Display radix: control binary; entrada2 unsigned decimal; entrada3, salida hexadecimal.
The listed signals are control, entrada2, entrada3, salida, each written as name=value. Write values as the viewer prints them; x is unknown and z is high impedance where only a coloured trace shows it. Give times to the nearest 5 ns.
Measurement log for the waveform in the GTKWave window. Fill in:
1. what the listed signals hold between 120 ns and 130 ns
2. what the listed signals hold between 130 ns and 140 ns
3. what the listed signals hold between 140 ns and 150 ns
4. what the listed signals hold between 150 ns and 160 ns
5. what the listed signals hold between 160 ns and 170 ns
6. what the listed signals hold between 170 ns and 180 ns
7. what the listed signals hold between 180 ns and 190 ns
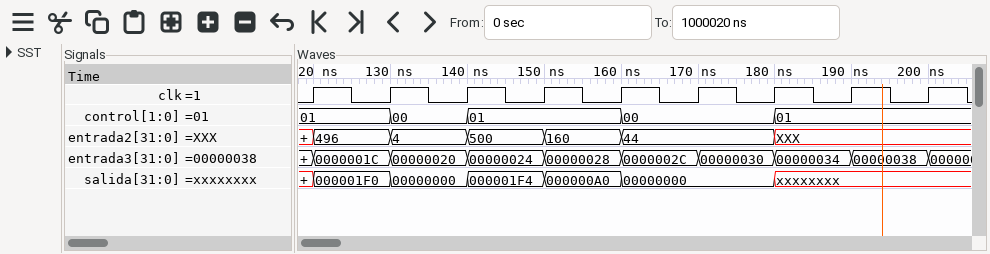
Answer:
control=01, entrada2=496, entrada3=0000001C, salida=000001F0
control=00, entrada2=4, entrada3=00000020, salida=00000000
control=01, entrada2=500, entrada3=00000024, salida=000001F4
control=01, entrada2=160, entrada3=00000028, salida=000000A0
control=00, entrada2=44, entrada3=0000002C, salida=00000000
control=00, entrada2=44, entrada3=00000030, salida=00000000
control=01, entrada2=XXX, entrada3=00000034, salida=xxxxxxxx
